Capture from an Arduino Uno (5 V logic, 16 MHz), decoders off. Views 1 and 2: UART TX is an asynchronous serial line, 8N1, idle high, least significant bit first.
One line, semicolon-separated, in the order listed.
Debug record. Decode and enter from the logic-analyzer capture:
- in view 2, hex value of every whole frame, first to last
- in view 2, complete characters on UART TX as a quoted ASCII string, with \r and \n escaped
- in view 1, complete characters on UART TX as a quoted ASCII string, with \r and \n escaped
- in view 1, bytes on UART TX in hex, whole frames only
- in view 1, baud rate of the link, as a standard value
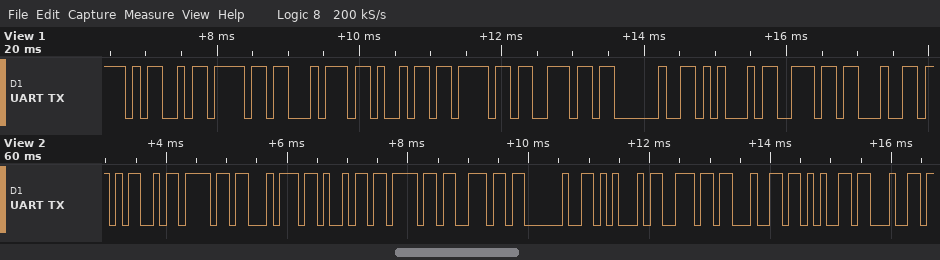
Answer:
4D 6F 74 69 6F 6E 20 45 6E 64 65 64; "Motion Ended"; "Motion End"; 0x4D 0x6F 0x74 0x69 0x6F 0x6E 0x20 0x45 0x6E 0x64; 9600 baud
